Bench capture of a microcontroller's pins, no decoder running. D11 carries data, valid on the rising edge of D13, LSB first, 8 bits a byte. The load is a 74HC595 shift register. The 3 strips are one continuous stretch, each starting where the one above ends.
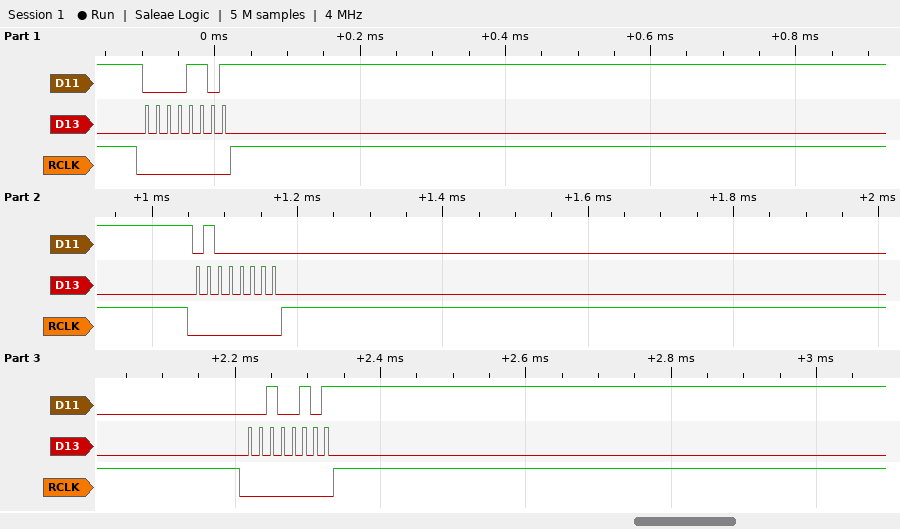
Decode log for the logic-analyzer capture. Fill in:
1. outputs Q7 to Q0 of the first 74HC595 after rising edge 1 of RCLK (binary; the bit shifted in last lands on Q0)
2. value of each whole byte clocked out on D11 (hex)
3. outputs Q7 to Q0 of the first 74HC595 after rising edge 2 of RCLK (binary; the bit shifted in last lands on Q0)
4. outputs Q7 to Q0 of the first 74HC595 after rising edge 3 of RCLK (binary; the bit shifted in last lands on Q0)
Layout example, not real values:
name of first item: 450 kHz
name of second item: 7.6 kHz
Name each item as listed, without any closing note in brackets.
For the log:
outputs Q7 to Q0 of the first 74HC595 after rising edge 1 of RCLK: 00001101
value of each whole byte clocked out on D11: B0 02 A4
outputs Q7 to Q0 of the first 74HC595 after rising edge 2 of RCLK: 01000000
outputs Q7 to Q0 of the first 74HC595 after rising edge 3 of RCLK: 00100101
